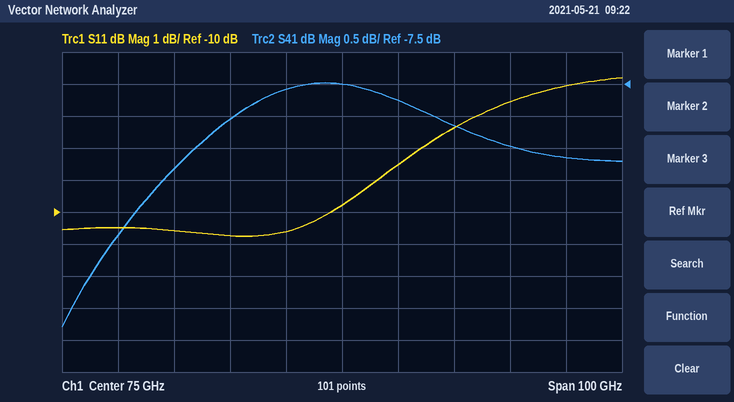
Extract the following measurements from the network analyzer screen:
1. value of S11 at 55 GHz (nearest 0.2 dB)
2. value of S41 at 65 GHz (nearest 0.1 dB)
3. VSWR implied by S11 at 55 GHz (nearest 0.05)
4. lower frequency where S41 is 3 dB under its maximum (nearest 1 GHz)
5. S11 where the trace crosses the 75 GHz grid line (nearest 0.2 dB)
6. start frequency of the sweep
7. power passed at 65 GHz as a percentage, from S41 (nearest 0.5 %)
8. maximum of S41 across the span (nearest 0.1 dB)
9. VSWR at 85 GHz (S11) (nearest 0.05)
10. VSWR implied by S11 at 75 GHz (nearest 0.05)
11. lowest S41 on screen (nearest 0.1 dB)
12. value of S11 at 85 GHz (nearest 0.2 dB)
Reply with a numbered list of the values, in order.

1. -10.8 dB
2. -7.6 dB
3. 1.80
4. 30 GHz
5. -9.8 dB
6. 25 GHz
7. 17.5 %
8. -7.5 dB
9. 2.20
10. 1.95
11. -11.3 dB
12. -8.6 dB
